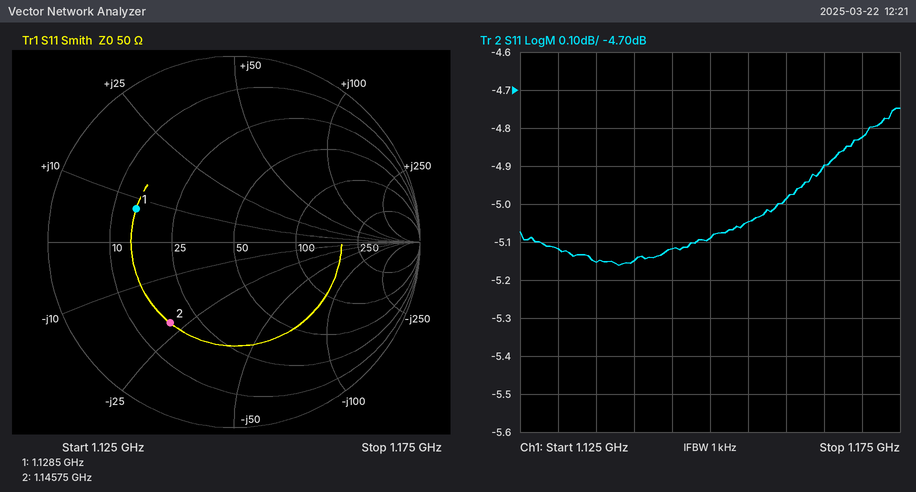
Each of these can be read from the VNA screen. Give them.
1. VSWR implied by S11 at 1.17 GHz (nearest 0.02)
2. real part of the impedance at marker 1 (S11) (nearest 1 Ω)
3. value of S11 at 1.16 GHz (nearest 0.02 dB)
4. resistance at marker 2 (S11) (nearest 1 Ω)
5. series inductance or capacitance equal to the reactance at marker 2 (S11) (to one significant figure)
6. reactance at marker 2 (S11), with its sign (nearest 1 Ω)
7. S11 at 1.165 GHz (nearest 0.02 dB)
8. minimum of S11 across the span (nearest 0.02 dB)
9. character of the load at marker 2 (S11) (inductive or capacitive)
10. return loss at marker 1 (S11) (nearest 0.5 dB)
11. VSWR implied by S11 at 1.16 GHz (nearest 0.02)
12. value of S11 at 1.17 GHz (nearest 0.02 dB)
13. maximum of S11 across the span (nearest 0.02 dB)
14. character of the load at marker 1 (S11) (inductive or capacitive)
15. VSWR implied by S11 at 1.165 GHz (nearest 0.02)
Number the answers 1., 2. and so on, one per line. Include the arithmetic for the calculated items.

1. |Γ| = 10^(-4.82/20) = 0.5741; VSWR = (1 + 0.5741)/(1 − 0.5741) ≈ 3.70
2. 15 Ω
3. -4.98 dB
4. 17 Ω
5. C = 1/(2π × 1.14575 GHz × 22 Ω) ≈ 6 pF
6. -22 Ω
7. -4.90 dB
8. -5.16 dB
9. capacitive
10. 5.0 dB
11. |Γ| = 10^(-4.98/20) = 0.5636; VSWR = (1 + 0.5636)/(1 − 0.5636) ≈ 3.58
12. -4.82 dB
13. -4.74 dB
14. inductive
15. |Γ| = 10^(-4.9/20) = 0.5689; VSWR = (1 + 0.5689)/(1 − 0.5689) ≈ 3.64
